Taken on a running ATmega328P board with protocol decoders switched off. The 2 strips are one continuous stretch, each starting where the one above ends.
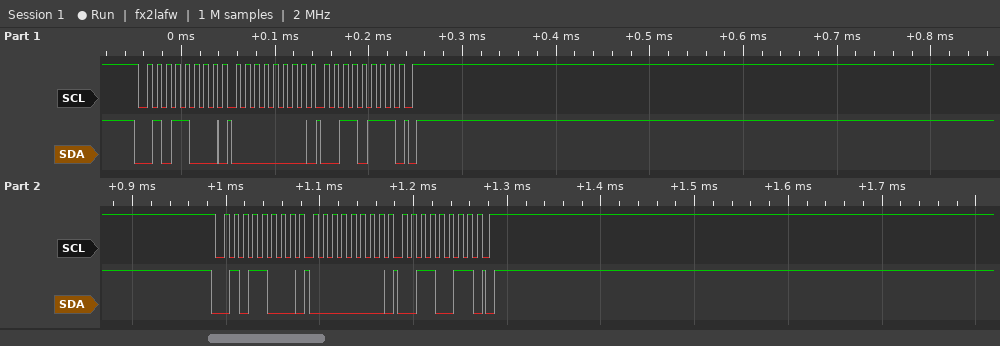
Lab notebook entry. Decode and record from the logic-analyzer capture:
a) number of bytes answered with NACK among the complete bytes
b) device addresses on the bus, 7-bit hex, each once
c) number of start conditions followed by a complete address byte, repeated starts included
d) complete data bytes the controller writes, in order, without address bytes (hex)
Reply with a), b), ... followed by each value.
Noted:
a) 0
b) 0x2C
c) 2
d) 00 37 00 33
